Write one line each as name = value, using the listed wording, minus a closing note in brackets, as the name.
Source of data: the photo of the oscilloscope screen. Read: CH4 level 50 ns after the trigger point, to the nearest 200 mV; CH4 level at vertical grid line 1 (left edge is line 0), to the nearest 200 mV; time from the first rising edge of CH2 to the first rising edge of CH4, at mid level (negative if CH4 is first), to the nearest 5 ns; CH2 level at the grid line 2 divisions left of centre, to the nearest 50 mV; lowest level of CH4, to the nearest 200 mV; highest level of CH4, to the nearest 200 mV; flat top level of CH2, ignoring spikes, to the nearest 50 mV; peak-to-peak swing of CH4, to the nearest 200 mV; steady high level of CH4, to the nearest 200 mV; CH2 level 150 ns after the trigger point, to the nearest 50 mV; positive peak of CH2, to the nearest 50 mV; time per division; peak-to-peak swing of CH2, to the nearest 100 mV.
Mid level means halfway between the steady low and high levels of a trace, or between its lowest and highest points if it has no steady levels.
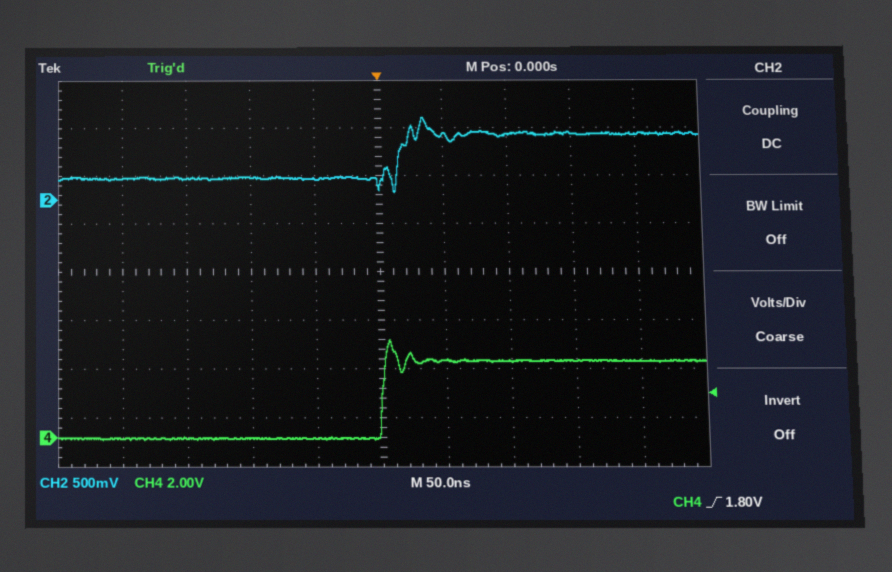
CH4 level 50 ns after the trigger point, to the nearest 200 mV = 3.2 V
CH4 level at vertical grid line 1 (left edge is line 0), to the nearest 200 mV = 0.0 V
time from the first rising edge of CH2 to the first rising edge of CH4, at mid level (negative if CH4 is first), to the nearest 5 ns = -15 ns
CH2 level at the grid line 2 divisions left of centre, to the nearest 50 mV = 250 mV
lowest level of CH4, to the nearest 200 mV = 0.0 V
highest level of CH4, to the nearest 200 mV = 4.0 V
flat top level of CH2, ignoring spikes, to the nearest 50 mV = 700 mV
peak-to-peak swing of CH4, to the nearest 200 mV = 4.0 V
steady high level of CH4, to the nearest 200 mV = 3.2 V
CH2 level 150 ns after the trigger point, to the nearest 50 mV = 700 mV
positive peak of CH2, to the nearest 50 mV = 850 mV
time per division = 50 ns
peak-to-peak swing of CH2, to the nearest 100 mV = 800 mV
